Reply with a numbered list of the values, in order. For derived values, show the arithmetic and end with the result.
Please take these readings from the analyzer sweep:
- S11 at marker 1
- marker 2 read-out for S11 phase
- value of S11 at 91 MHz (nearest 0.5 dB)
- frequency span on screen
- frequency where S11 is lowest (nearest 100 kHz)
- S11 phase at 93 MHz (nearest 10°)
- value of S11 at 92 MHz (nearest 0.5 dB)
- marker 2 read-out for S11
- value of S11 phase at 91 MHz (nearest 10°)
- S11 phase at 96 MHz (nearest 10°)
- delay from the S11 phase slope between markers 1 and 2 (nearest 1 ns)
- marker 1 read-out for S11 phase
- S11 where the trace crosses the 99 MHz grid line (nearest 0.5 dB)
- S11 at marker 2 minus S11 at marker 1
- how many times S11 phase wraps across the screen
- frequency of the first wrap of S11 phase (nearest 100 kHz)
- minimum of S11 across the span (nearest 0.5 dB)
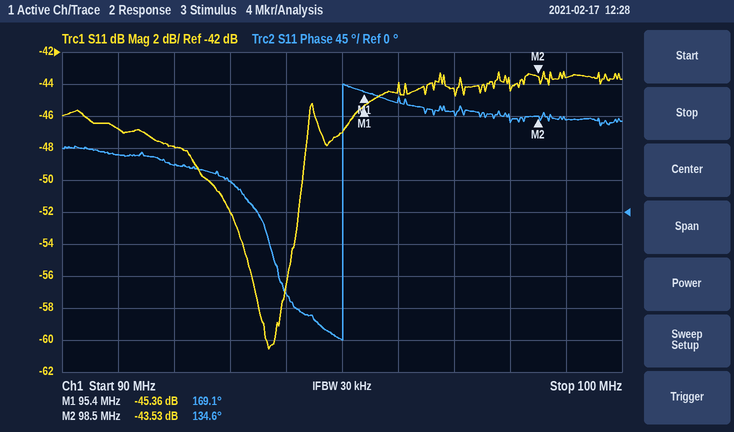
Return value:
1. -45.36 dB
2. 134.6°
3. -47.0 dB
4. 10 MHz
5. 93.7 MHz
6. 40°
7. -48.0 dB
8. -43.53 dB
9. 80°
10. 160°
11. −(134.6° − (169.1°))/(360° × 3.1 MHz) ≈ 31 ns
12. 169.1°
13. -43.5 dB
14. -43.53 − (-45.36) = 1.83 dB
15. 1
16. 95.0 MHz
17. -60.5 dB
